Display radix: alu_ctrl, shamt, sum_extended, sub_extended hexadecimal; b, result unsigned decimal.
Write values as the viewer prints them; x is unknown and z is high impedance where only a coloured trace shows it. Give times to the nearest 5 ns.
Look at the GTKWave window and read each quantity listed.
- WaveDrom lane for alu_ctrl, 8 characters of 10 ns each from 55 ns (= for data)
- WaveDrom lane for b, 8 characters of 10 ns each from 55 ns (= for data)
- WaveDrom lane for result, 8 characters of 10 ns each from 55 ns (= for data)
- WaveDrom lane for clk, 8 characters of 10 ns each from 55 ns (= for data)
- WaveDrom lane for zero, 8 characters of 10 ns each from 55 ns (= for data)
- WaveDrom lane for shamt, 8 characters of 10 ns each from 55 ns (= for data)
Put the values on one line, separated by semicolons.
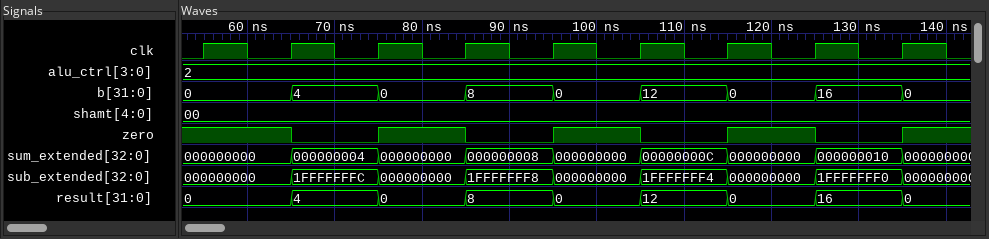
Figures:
{name: 'alu_ctrl', wave: '=.......', data: '2'}; {name: 'b', wave: '========', data: '0 4 0 8 0 12 0 16'}; {name: 'result', wave: '========', data: '0 4 0 8 0 12 0 16'}; {name: 'clk', wave: 'p.......'}; {name: 'zero', wave: '10101010'}; {name: 'shamt', wave: '=.......', data: '00'}
